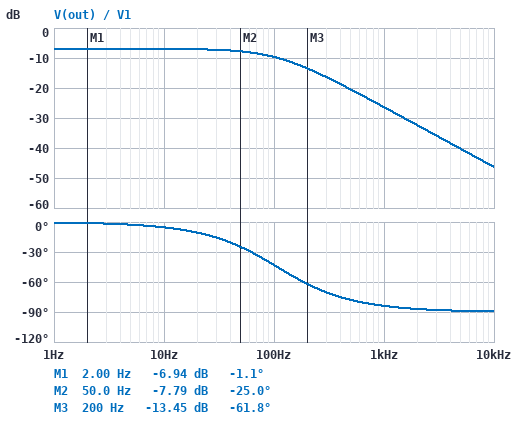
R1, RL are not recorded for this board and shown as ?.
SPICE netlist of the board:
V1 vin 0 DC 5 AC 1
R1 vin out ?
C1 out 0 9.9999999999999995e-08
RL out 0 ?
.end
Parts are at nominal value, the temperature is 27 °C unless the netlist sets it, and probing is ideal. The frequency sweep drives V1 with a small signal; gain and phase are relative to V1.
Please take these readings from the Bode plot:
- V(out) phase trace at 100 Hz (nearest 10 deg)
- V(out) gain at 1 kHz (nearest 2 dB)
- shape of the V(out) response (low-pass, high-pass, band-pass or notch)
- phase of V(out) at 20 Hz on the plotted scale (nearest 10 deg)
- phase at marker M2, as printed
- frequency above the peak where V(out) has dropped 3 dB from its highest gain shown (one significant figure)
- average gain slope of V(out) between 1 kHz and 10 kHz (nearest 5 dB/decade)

-40 deg
-26 dB
low-pass
-10 deg
-25.0 deg
100 Hz
-20 dB/decade
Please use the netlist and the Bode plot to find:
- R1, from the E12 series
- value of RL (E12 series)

33 kΩ
27 kΩ
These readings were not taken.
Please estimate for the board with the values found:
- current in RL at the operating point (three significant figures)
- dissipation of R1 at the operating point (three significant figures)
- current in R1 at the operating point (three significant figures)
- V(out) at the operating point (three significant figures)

83.3 µA
229 µW
83.3 µA
2.25 V
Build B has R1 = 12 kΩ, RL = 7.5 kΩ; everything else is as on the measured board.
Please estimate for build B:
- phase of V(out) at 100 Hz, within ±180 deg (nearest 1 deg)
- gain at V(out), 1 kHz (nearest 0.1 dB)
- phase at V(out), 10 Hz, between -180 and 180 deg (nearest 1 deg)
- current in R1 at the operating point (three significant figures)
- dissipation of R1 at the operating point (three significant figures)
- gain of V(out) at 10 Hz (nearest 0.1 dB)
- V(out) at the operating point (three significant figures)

-16 deg
-18.0 dB
-2 deg
256 µA
789 µW
-8.3 dB
1.92 V
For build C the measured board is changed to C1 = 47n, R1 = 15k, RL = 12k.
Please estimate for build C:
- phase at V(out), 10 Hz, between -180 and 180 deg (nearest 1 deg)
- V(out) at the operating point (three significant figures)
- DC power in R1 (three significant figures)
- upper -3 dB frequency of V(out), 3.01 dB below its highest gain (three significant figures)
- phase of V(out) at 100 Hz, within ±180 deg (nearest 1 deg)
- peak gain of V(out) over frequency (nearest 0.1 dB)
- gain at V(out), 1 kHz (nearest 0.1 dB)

-1 deg
2.22 V
514 µW
508 Hz
-11 deg
-7.0 dB
-13.9 dB
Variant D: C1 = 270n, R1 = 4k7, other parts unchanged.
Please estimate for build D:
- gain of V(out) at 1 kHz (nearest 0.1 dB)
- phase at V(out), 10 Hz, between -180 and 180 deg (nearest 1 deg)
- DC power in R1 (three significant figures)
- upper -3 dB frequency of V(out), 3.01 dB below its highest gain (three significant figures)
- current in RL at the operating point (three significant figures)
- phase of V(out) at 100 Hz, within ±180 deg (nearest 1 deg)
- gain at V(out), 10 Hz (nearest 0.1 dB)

-18.1 dB
-4 deg
117 µW
147 Hz
158 µA
-34 deg
-1.4 dB
